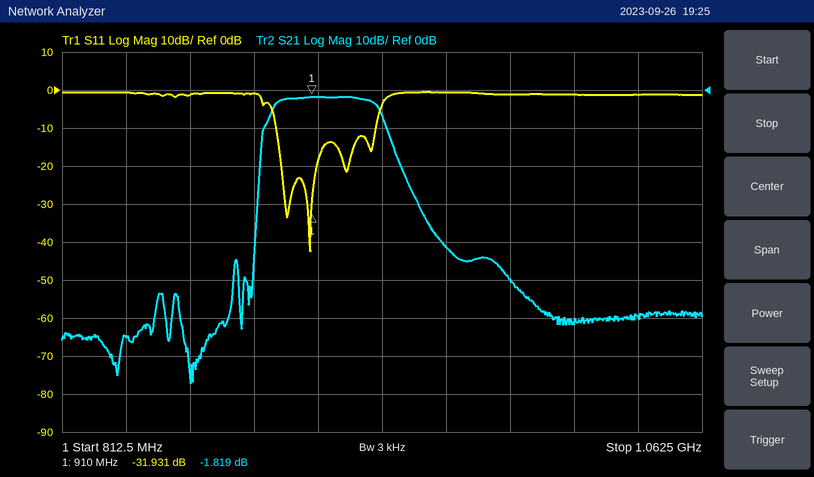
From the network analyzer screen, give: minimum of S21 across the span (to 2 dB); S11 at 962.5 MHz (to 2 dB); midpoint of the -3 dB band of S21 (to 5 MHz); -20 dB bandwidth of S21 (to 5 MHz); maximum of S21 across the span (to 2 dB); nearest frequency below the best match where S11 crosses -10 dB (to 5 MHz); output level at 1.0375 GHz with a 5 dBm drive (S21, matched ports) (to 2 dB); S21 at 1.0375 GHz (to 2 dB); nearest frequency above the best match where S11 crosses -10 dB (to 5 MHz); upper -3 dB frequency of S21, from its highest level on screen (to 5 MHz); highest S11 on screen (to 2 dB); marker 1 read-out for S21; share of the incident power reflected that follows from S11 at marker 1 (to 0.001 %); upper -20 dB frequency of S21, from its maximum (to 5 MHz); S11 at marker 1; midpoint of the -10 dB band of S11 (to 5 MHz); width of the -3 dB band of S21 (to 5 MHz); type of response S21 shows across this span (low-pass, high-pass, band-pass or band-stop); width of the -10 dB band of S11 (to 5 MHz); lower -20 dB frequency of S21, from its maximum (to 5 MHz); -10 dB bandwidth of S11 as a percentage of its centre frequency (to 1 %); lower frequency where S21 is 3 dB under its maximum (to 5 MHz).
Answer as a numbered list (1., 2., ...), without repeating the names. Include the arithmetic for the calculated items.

1. -78 dB
2. 0 dB
3. 915 MHz
4. 945 MHz − 890 MHz = 55 MHz
5. -2 dB
6. 895 MHz
7. 5 dBm + (-60 dB) = -54 dBm
8. -60 dB
9. 935 MHz
10. 935 MHz
11. 0 dB
12. -1.819 dB
13. 10^(-31.931/10) ≈ 0.064 %
14. 945 MHz
15. -31.931 dB
16. 915 MHz
17. 935 MHz − 895 MHz = 40 MHz
18. band-pass
19. 935 MHz − 895 MHz = 40 MHz
20. 890 MHz
21. 40 MHz / 915 MHz ≈ 4 %
22. 895 MHz
